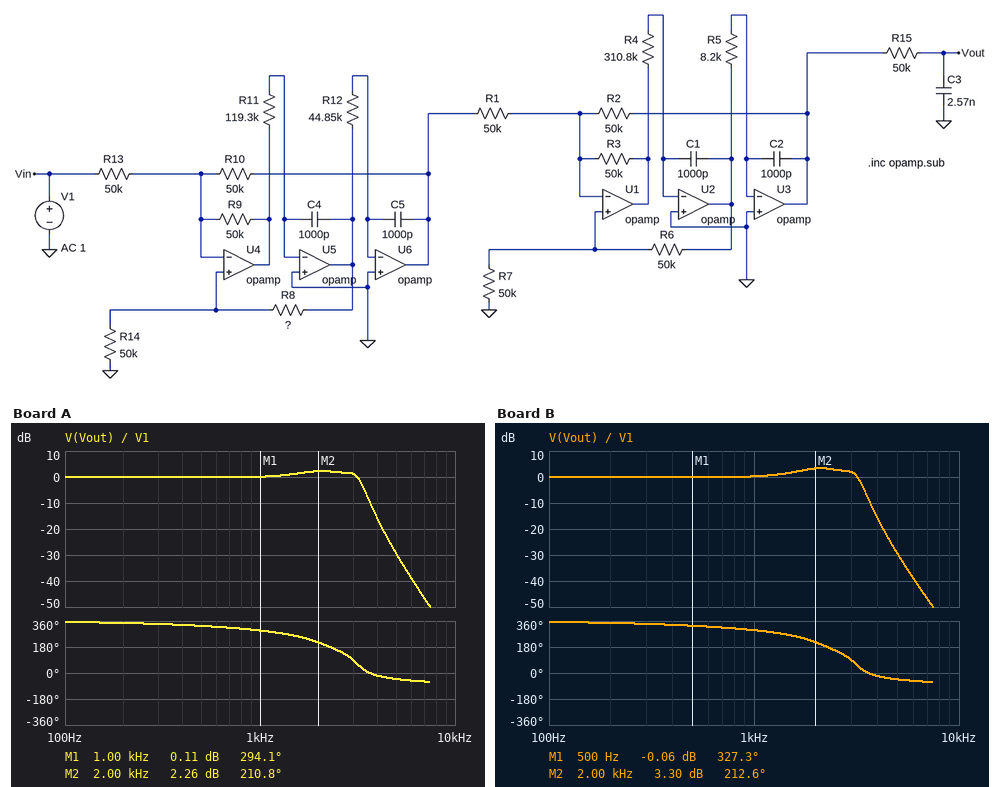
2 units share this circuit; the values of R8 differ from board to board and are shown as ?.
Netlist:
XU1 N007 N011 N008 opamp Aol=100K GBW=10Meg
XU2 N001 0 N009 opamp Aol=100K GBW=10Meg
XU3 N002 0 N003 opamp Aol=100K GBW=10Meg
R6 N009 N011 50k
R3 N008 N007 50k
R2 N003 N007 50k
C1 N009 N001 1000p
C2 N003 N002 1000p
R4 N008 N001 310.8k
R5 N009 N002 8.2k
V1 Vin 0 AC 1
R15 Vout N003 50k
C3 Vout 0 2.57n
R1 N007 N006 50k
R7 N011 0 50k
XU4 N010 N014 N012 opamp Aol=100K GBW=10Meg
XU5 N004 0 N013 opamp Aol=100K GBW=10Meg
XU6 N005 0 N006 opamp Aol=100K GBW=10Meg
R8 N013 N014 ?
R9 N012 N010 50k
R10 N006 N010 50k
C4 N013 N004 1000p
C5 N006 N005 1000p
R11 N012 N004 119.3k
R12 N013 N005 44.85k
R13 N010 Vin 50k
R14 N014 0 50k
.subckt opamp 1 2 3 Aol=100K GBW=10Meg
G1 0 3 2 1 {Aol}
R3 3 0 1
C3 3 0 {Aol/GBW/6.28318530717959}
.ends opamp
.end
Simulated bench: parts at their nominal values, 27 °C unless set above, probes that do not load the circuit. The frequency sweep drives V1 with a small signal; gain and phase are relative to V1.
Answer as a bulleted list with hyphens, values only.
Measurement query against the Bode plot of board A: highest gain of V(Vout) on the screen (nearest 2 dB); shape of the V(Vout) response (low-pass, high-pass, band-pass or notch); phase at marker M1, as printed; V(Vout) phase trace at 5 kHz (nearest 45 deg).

- 2 dB
- low-pass
- 294.1 deg
- -45 deg
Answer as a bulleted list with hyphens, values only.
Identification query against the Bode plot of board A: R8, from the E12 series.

- 82 kΩ
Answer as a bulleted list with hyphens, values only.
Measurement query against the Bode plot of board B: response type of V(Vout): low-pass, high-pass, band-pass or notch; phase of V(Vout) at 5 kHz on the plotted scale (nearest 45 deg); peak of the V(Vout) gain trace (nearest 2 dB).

- low-pass
- -45 deg
- 4 dB
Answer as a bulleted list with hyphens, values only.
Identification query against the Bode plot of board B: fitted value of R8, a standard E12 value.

- 100 kΩ
